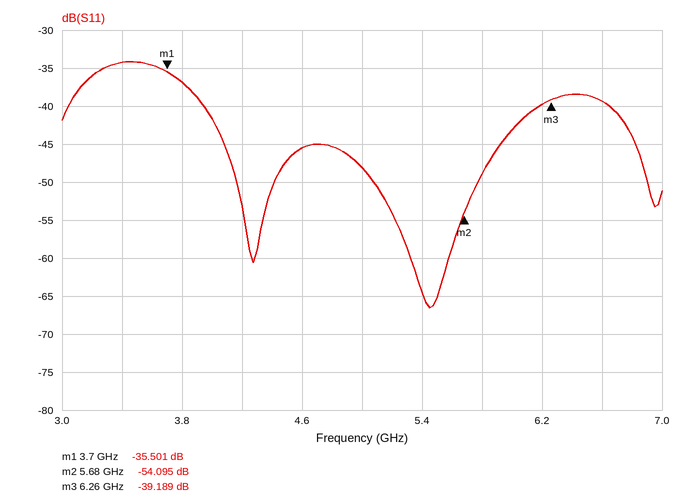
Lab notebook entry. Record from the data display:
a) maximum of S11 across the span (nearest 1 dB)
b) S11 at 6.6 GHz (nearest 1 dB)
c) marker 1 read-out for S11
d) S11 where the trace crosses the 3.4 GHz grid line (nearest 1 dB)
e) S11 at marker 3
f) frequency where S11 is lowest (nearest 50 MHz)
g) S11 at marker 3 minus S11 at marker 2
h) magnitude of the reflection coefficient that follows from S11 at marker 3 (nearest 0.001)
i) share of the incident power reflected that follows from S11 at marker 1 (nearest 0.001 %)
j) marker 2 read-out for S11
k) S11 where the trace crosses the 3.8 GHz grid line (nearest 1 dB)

-34 dB
-39 dB
-35.501 dB
-34 dB
-39.189 dB
5.45 GHz
14.906 dB
0.011
0.028 %
-54.095 dB
-37 dB
